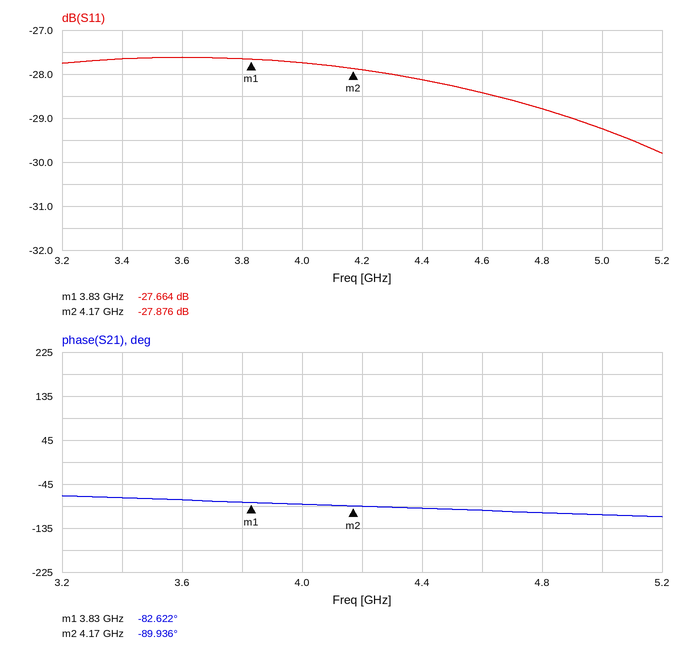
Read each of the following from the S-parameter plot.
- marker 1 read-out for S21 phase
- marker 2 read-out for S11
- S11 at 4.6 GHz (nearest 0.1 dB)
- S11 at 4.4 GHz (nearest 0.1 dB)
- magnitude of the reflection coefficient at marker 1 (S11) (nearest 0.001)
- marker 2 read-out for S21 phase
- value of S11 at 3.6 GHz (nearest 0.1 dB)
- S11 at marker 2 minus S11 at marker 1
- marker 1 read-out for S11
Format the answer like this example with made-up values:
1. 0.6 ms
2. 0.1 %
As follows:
1. -82.622°
2. -27.876 dB
3. -28.4 dB
4. -28.1 dB
5. 0.041
6. -89.936°
7. -27.6 dB
8. -0.212 dB
9. -27.664 dB
